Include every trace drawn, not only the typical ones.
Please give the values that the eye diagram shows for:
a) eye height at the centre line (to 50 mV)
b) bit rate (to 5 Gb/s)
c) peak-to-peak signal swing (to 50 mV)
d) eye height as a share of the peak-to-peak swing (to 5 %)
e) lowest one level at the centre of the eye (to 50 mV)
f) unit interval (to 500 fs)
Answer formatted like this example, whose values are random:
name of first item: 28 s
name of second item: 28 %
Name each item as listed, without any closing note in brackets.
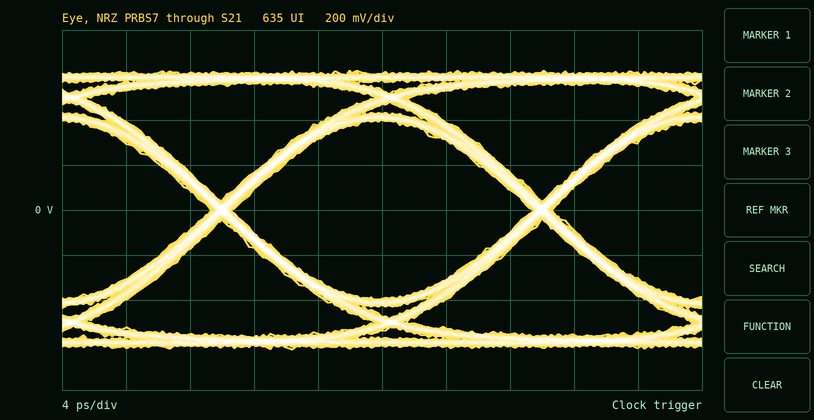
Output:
eye height at the centre line: 800 mV
bit rate: 50 Gb/s
peak-to-peak signal swing: 1.25 V
eye height as a share of the peak-to-peak swing: 65 %
lowest one level at the centre of the eye: 400 mV
unit interval: 20.0 ps
